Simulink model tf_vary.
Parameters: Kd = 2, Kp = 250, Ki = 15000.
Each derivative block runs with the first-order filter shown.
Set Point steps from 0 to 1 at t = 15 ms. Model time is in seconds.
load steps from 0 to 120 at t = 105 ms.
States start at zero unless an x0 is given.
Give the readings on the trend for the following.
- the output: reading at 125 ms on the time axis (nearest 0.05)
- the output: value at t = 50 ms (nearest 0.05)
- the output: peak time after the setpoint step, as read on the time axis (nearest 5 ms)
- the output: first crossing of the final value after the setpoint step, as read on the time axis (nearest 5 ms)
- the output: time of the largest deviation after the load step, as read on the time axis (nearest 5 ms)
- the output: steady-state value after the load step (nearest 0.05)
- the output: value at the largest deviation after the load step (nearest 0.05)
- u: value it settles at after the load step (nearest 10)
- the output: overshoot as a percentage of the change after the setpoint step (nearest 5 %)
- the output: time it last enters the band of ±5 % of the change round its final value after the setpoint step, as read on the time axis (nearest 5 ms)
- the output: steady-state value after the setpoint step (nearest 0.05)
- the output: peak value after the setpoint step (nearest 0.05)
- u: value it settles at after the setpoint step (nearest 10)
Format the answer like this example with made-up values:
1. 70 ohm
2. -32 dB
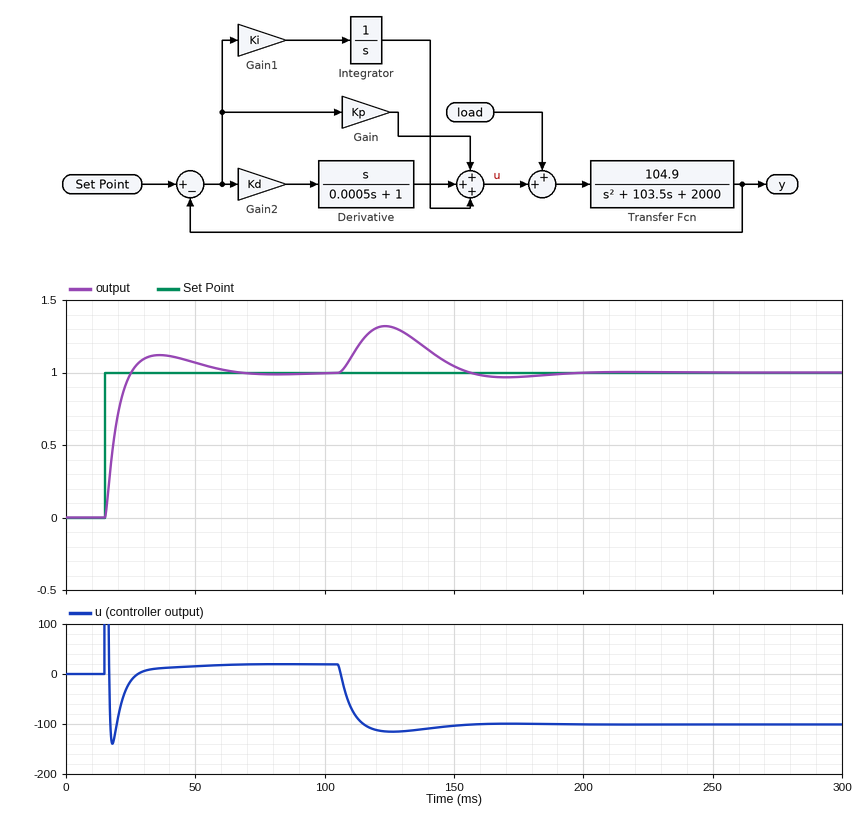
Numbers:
1. 1.30
2. 1.05
3. 35 ms
4. 25 ms
5. 125 ms
6. 1.00
7. 1.30
8. -100
9. 10 %
10. 55 ms
11. 1.00
12. 1.10
13. 20
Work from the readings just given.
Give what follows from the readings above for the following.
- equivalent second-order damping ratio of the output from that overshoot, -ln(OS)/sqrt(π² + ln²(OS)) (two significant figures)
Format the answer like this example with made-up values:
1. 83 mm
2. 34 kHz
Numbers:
1. 0.59
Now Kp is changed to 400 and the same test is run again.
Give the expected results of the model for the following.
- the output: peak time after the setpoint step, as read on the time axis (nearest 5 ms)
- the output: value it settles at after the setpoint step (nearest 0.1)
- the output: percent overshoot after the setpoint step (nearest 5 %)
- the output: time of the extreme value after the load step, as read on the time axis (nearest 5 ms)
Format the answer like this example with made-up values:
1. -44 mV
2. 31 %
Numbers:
1. 30 ms
2. 1.0
3. 15 %
4. 120 ms
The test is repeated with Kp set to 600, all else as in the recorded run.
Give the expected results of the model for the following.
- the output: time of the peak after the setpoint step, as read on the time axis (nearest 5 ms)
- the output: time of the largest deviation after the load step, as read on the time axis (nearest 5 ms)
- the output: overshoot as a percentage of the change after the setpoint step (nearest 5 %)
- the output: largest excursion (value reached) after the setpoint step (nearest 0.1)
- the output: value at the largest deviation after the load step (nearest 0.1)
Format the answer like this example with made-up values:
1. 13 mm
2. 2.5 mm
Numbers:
1. 25 ms
2. 120 ms
3. 20 %
4. 1.2
5. 1.2
